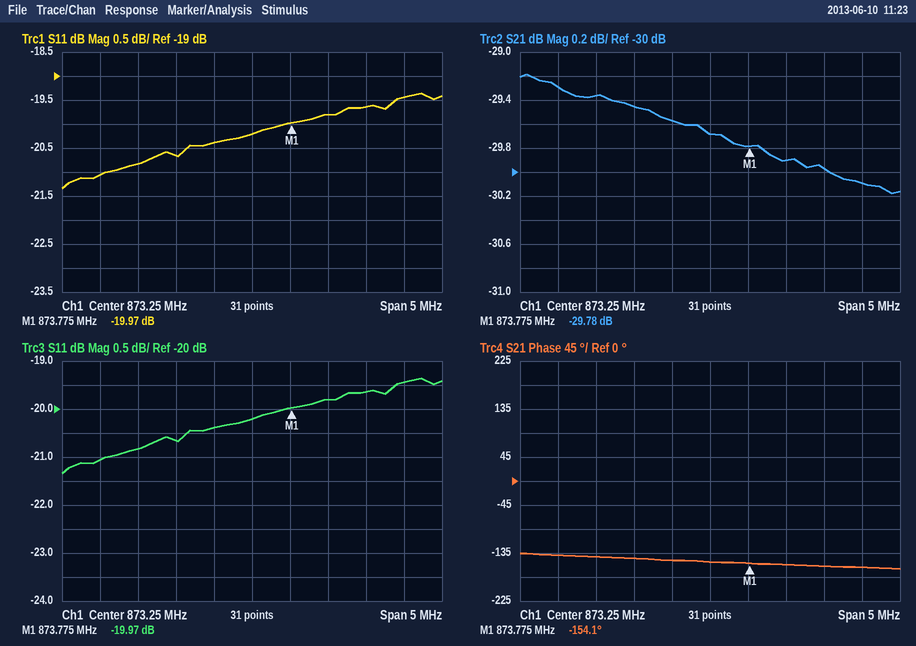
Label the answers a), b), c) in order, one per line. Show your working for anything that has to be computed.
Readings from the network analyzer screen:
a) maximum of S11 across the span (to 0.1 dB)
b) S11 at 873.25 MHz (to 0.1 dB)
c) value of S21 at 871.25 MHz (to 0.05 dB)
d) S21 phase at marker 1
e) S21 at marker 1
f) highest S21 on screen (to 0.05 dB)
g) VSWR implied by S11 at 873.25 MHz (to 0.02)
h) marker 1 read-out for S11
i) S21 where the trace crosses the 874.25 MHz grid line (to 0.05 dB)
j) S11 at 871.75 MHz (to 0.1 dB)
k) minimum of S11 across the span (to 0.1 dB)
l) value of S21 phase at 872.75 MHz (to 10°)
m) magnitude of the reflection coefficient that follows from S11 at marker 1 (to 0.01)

a) -19.4 dB
b) -20.2 dB
c) -29.30 dB
d) -154.1°
e) -29.78 dB
f) -29.20 dB
g) |Γ| = 10^(-20.2/20) = 0.0977; VSWR = (1 + 0.0977)/(1 − 0.0977) ≈ 1.22
h) -19.97 dB
i) -29.90 dB
j) -20.8 dB
k) -21.3 dB
l) -150°
m) 10^(-19.97/20) ≈ 0.10
